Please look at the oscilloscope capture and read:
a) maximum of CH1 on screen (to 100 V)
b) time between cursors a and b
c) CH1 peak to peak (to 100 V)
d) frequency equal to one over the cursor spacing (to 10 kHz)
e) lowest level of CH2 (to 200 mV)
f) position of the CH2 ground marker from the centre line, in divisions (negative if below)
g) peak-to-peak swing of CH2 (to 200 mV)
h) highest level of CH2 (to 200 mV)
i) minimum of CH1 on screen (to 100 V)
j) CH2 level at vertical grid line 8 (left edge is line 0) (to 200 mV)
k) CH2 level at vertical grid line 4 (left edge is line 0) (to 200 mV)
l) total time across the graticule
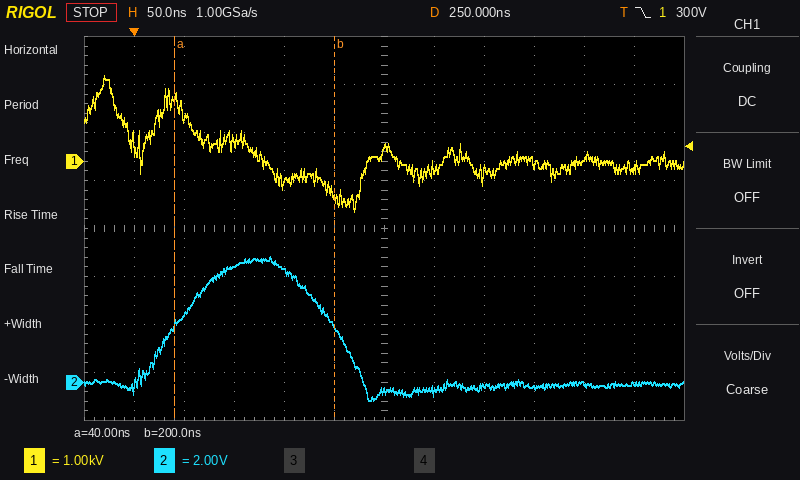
1.8 kV
160 ns
2.8 kV
6.25 MHz
-800 mV
-3.2 div
6.0 V
5.2 V
-1.0 kV
-200 mV
4.6 V
600 ns
